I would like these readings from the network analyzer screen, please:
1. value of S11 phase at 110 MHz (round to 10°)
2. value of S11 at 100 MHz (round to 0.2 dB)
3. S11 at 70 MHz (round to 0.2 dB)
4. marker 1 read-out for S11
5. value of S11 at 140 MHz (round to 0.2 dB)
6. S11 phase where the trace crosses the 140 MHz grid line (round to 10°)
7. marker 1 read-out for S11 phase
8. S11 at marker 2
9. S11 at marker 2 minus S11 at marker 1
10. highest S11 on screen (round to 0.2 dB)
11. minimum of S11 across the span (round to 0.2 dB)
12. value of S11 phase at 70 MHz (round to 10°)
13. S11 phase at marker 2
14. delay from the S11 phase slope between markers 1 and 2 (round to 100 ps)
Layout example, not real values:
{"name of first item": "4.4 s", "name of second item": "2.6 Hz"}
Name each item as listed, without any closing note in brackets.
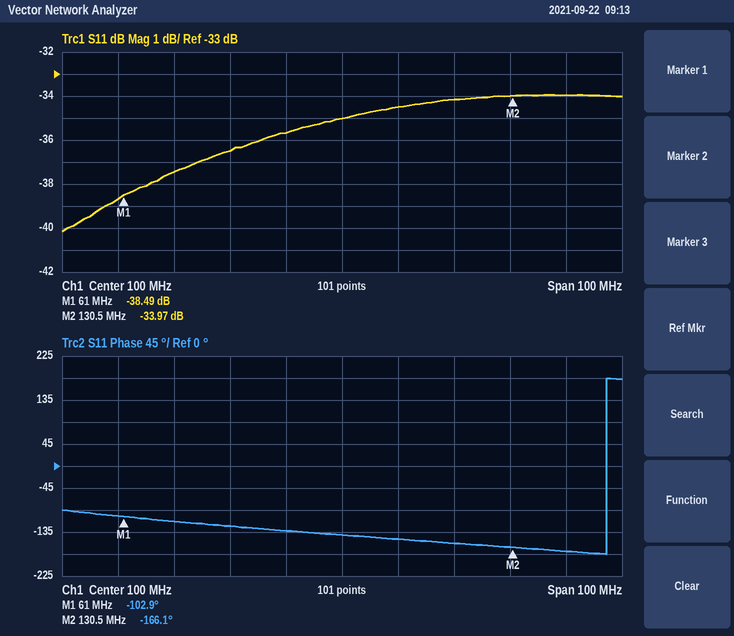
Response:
{"value of S11 phase at 110 MHz": "-150°", "value of S11 at 100 MHz": "-35.0 dB", "S11 at 70 MHz": "-37.4 dB", "marker 1 read-out for S11": "-38.49 dB", "value of S11 at 140 MHz": "-34.0 dB", "S11 phase where the trace crosses the 140 MHz grid line": "-170°", "marker 1 read-out for S11 phase": "-102.9°", "S11 at marker 2": "-33.97 dB", "S11 at marker 2 minus S11 at marker 1": "4.52 dB", "highest S11 on screen": "-34.0 dB", "minimum of S11 across the span": "-40.2 dB", "value of S11 phase at 70 MHz": "-110°", "S11 phase at marker 2": "-166.1°", "delay from the S11 phase slope between markers 1 and 2": "2.5 ns"}
